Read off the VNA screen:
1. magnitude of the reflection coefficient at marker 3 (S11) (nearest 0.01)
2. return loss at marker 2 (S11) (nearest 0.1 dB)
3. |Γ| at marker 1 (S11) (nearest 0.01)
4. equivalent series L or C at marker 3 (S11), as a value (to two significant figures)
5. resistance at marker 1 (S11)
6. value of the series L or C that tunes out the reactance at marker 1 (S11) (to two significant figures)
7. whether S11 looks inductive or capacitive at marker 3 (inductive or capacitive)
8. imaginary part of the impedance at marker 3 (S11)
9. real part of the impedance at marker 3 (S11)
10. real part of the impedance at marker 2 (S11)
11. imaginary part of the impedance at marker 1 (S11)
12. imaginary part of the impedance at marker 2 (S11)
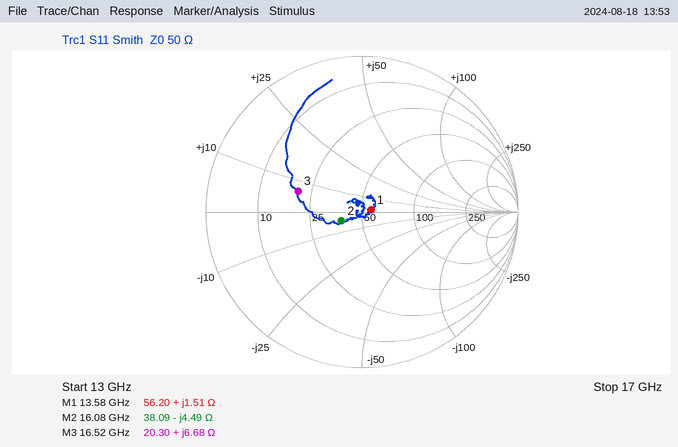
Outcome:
0.43
16.8 dB
0.06
64 pH
56.20 Ω
7.8 pF
inductive
+6.68 Ω
20.30 Ω
38.09 Ω
+1.51 Ω
-4.49 Ω
